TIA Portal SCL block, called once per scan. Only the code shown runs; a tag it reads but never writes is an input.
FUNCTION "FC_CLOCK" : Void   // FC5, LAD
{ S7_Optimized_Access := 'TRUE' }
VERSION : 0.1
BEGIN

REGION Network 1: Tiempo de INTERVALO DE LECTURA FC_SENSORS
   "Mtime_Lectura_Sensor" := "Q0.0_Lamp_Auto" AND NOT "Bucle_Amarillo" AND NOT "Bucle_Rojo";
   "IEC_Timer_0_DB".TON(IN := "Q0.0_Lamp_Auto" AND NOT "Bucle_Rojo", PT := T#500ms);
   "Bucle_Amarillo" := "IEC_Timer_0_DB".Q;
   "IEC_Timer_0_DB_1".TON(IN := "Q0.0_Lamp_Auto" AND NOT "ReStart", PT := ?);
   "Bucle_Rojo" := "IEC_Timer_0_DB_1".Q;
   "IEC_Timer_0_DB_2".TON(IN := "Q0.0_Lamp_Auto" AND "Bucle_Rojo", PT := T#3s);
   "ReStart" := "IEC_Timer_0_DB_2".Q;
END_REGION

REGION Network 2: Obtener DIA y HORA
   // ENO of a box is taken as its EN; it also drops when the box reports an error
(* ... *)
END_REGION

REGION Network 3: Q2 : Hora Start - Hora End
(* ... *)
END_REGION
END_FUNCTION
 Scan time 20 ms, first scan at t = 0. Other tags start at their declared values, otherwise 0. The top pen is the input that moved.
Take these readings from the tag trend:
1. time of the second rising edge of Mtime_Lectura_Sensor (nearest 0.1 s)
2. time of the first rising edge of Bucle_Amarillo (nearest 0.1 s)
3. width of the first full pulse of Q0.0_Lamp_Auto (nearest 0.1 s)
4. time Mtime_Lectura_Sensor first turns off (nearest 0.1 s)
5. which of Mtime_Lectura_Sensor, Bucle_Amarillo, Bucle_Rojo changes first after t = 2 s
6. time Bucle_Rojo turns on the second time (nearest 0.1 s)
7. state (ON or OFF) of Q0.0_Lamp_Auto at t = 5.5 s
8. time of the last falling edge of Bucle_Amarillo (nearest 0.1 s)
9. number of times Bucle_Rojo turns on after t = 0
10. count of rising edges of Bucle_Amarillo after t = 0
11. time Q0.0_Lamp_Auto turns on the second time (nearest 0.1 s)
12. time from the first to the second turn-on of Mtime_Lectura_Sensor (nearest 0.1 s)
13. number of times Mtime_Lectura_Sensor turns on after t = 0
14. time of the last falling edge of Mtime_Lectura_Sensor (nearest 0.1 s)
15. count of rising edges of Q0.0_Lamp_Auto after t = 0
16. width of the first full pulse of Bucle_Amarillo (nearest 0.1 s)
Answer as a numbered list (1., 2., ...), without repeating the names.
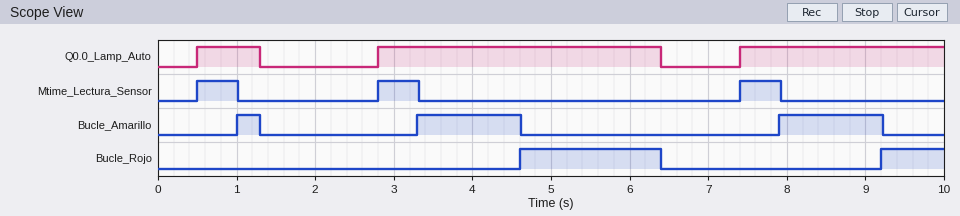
1. 2.8 s
2. 1.0 s
3. 0.8 s
4. 1.0 s
5. Mtime_Lectura_Sensor
6. 9.2 s
7. ON
8. 9.2 s
9. 2
10. 3
11. 2.8 s
12. 2.3 s
13. 3
14. 7.9 s
15. 3
16. 0.3 s
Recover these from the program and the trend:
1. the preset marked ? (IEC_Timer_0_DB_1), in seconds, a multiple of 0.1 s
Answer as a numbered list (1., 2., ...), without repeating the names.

1. 1.8 s
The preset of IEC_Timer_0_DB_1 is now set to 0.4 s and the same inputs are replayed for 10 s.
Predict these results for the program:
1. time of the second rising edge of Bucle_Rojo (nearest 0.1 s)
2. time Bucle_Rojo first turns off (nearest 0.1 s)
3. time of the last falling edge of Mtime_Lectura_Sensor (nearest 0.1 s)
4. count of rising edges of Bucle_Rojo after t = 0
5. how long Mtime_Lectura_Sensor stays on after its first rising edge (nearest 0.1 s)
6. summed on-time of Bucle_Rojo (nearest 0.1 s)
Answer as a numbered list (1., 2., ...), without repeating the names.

1. 3.2 s
2. 1.3 s
3. 7.8 s
4. 3
5. 0.4 s
6. 5.6 s
